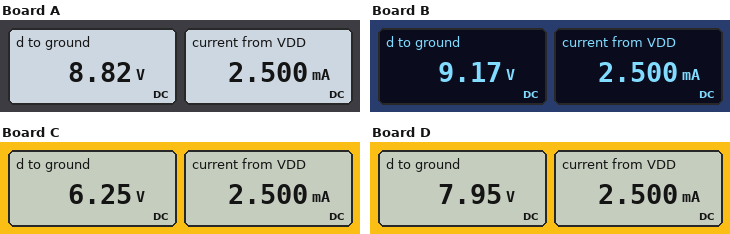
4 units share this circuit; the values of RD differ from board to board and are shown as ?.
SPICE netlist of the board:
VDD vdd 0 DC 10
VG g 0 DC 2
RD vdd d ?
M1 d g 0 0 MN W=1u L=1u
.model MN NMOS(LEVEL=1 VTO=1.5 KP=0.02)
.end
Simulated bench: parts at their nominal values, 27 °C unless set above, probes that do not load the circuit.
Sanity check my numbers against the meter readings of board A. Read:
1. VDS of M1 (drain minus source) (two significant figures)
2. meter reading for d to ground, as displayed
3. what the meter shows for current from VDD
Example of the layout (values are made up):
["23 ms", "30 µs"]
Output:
["8.8 V", "8.82 V", "2.500 mA"]
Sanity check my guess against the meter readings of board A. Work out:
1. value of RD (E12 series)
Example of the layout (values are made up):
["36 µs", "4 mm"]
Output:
["470 Ω"]
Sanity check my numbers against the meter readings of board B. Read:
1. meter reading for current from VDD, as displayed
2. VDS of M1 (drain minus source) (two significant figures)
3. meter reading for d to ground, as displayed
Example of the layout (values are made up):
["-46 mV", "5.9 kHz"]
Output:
["2.500 mA", "9.2 V", "9.17 V"]
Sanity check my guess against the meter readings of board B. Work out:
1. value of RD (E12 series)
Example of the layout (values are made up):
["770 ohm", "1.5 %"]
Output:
["330 Ω"]
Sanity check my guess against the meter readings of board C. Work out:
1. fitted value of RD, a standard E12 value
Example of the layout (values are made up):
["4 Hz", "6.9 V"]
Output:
["1.5 kΩ"]
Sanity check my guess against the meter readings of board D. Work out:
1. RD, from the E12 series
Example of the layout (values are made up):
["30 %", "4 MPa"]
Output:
["820 Ω"]
